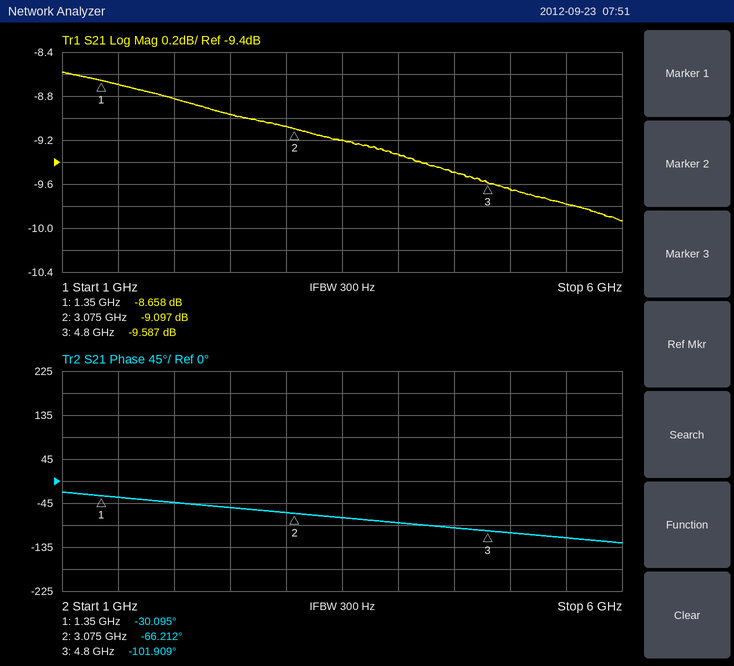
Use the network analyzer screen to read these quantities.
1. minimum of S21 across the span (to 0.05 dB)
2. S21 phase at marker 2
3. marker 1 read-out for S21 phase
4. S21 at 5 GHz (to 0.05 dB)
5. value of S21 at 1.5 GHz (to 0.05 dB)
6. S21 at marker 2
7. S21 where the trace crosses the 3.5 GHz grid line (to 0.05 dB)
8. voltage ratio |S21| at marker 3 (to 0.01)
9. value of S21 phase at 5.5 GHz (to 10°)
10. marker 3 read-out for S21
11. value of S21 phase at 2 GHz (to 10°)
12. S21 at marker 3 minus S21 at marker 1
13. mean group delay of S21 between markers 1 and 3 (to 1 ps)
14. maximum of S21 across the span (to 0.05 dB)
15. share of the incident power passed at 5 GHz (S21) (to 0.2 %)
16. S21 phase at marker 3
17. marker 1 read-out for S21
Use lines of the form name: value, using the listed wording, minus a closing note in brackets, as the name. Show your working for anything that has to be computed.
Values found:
minimum of S21 across the span: -9.95 dB
S21 phase at marker 2: -66.212°
marker 1 read-out for S21 phase: -30.095°
S21 at 5 GHz: -9.65 dB
value of S21 at 1.5 GHz: -8.70 dB
S21 at marker 2: -9.097 dB
S21 where the trace crosses the 3.5 GHz grid line: -9.20 dB
voltage ratio |S21| at marker 3: 10^(-9.587/20) ≈ 0.33
value of S21 phase at 5.5 GHz: -120°
marker 3 read-out for S21: -9.587 dB
value of S21 phase at 2 GHz: -40°
S21 at marker 3 minus S21 at marker 1: -9.587 − (-8.658) = -0.929 dB
mean group delay of S21 between markers 1 and 3: −(-101.909° − (-30.095°))/(360° × 3.45 GHz) ≈ 58 ps
maximum of S21 across the span: -8.60 dB
share of the incident power passed at 5 GHz (S21): 10^(-9.65/10) ≈ 10.8 %
S21 phase at marker 3: -101.909°
marker 1 read-out for S21: -8.658 dB
